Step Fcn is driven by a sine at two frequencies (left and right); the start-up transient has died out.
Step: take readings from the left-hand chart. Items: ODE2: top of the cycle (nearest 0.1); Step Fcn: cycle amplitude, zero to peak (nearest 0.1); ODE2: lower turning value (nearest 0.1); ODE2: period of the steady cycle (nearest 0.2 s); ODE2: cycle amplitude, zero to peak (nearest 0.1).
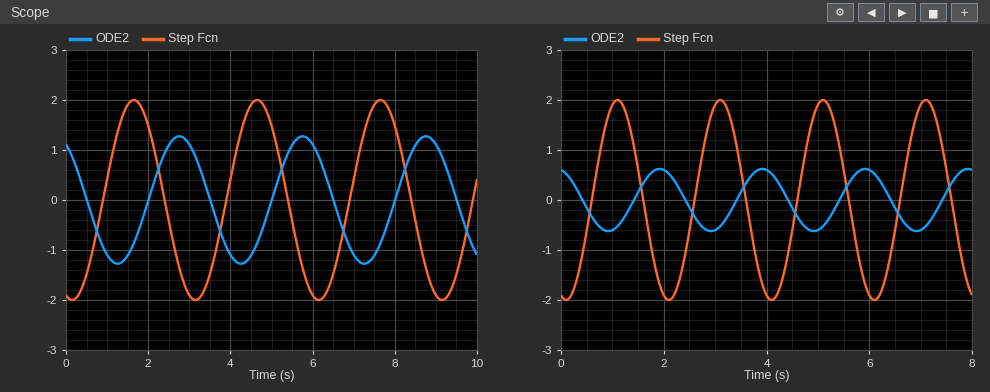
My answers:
1.3
2.0
-1.3
3.0 s
1.3
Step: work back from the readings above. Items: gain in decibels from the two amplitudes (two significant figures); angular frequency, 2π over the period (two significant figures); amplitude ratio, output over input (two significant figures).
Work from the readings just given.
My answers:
-3.7 dB
2.1 rad/s
0.65
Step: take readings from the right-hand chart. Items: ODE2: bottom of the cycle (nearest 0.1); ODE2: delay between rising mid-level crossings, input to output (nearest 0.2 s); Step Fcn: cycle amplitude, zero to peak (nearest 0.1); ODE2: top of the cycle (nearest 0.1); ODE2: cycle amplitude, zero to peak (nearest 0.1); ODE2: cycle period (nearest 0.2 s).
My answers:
-0.6
0.8 s
2.0
0.6
0.6
2.0 s
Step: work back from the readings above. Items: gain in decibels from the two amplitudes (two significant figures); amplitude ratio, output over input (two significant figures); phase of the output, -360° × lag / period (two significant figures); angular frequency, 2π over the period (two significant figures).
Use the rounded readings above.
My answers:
-10 dB
0.30
-140°
3.1 rad/s
